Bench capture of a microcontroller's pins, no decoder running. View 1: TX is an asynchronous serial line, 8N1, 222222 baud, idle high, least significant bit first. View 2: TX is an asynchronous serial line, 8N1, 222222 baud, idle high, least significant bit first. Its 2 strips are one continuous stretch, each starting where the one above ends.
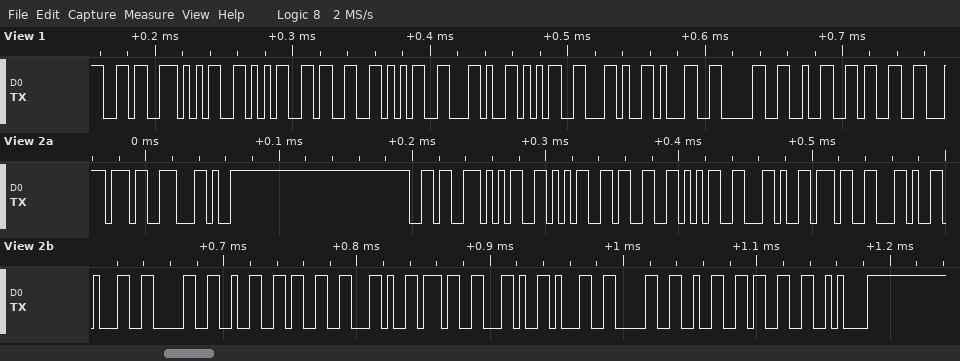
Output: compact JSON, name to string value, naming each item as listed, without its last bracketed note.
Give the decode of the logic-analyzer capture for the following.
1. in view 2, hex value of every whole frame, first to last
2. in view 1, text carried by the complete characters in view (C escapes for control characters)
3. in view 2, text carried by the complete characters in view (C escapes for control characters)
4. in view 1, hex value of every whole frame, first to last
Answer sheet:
{"in view 2, hex value of every whole frame, first to last": "37 2C 36 35 35 33 35 2C 37 2C 31 30 32 33 2C 37 2C 31 30 32 33 0A", "in view 1, text carried by the complete characters in view": "\"65535,5,1023\"", "in view 2, text carried by the complete characters in view": "\"7,65535,7,1023,7,1023\\n\"", "in view 1, hex value of every whole frame, first to last": "36 35 35 33 35 2C 35 2C 31 30 32 33"}
